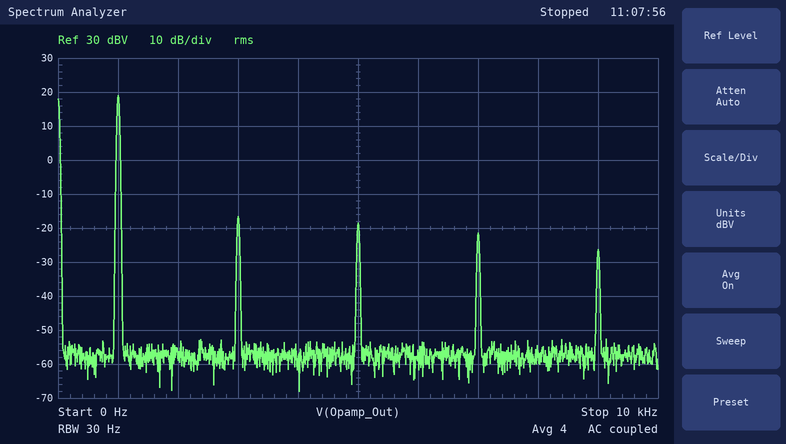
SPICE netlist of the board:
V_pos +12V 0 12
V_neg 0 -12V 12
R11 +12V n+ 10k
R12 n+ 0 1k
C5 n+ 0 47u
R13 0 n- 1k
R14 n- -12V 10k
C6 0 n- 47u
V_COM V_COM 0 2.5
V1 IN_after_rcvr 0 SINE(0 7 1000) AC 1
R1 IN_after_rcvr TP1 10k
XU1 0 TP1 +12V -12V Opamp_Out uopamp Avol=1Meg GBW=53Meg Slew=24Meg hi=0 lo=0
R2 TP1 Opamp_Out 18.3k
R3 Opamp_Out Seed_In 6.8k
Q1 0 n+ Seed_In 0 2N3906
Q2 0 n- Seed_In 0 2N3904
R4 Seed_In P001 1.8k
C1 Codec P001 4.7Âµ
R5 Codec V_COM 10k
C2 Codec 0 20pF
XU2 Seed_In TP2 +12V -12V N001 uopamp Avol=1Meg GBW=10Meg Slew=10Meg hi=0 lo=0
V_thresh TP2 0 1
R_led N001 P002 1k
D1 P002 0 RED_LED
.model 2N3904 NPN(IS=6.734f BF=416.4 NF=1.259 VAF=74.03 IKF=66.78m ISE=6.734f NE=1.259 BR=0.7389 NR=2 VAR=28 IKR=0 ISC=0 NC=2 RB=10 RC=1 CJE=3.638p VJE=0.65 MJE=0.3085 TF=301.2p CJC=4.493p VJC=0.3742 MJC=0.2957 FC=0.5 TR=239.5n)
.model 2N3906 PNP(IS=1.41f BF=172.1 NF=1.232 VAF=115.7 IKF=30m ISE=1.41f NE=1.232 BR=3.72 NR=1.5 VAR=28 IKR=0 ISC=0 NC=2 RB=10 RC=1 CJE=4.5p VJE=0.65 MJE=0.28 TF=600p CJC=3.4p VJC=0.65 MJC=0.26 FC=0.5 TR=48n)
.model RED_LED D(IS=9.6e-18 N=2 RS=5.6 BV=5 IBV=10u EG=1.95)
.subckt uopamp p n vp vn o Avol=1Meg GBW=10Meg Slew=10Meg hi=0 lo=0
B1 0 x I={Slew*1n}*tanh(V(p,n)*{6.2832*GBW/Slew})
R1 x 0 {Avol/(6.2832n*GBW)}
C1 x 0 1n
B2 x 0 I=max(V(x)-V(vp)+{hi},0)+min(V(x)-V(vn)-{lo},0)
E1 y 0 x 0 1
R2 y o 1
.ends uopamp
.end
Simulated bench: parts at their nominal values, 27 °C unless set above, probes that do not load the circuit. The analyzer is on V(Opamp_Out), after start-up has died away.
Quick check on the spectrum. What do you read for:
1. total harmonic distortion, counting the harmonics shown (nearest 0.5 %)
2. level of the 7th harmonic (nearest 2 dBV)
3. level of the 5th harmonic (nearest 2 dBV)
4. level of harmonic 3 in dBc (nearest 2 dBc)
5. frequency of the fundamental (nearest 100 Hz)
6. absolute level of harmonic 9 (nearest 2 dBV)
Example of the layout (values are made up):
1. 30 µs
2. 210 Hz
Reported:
1. 2.5 %
2. -22 dBV
3. -18 dBV
4. -36 dBc
5. 1.0 kHz
6. -26 dBV
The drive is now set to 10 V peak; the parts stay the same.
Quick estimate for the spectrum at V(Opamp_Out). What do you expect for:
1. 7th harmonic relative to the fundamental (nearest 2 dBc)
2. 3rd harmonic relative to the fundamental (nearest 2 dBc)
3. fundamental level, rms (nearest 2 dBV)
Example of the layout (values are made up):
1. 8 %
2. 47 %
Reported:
1. -32 dBc
2. -16 dBc
3. 20 dBV
